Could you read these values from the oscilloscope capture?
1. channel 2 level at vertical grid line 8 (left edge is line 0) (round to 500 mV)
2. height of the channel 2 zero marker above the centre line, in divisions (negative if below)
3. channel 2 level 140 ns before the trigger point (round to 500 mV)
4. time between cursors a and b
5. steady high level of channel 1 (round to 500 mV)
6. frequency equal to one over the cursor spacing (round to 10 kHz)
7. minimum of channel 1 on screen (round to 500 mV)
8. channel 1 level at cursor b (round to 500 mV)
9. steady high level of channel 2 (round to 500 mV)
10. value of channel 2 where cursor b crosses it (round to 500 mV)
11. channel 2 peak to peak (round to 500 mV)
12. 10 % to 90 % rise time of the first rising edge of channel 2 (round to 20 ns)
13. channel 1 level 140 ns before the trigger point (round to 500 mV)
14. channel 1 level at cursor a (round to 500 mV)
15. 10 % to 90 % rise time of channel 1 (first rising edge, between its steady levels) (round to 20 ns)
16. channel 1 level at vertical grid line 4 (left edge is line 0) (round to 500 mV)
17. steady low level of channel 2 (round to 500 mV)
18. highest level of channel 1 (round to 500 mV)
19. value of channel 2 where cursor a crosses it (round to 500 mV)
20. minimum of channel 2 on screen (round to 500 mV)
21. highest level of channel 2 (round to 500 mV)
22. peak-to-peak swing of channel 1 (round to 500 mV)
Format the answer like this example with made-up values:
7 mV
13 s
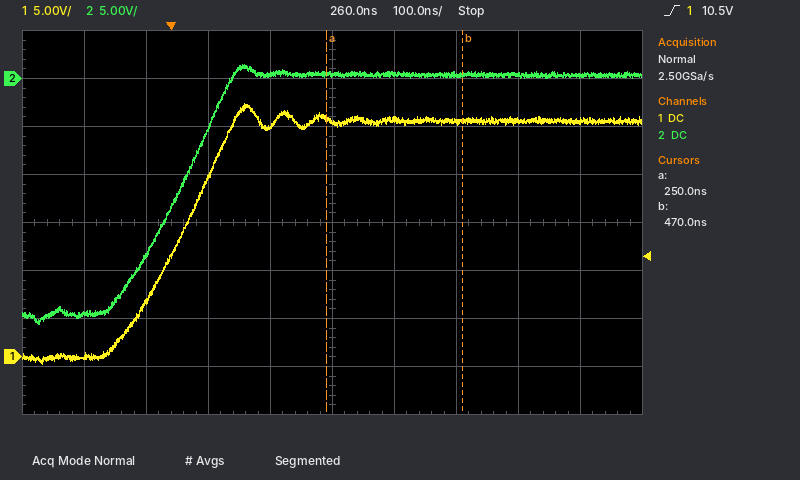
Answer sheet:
500 mV
+3.0 div
-24.5 V
220 ns
24.5 V
4.55 MHz
-500 mV
24.5 V
500 mV
500 mV
27.0 V
160 ns
0.0 V
25.0 V
160 ns
24.0 V
-24.5 V
26.5 V
500 mV
-25.5 V
1.5 V
27.0 V
